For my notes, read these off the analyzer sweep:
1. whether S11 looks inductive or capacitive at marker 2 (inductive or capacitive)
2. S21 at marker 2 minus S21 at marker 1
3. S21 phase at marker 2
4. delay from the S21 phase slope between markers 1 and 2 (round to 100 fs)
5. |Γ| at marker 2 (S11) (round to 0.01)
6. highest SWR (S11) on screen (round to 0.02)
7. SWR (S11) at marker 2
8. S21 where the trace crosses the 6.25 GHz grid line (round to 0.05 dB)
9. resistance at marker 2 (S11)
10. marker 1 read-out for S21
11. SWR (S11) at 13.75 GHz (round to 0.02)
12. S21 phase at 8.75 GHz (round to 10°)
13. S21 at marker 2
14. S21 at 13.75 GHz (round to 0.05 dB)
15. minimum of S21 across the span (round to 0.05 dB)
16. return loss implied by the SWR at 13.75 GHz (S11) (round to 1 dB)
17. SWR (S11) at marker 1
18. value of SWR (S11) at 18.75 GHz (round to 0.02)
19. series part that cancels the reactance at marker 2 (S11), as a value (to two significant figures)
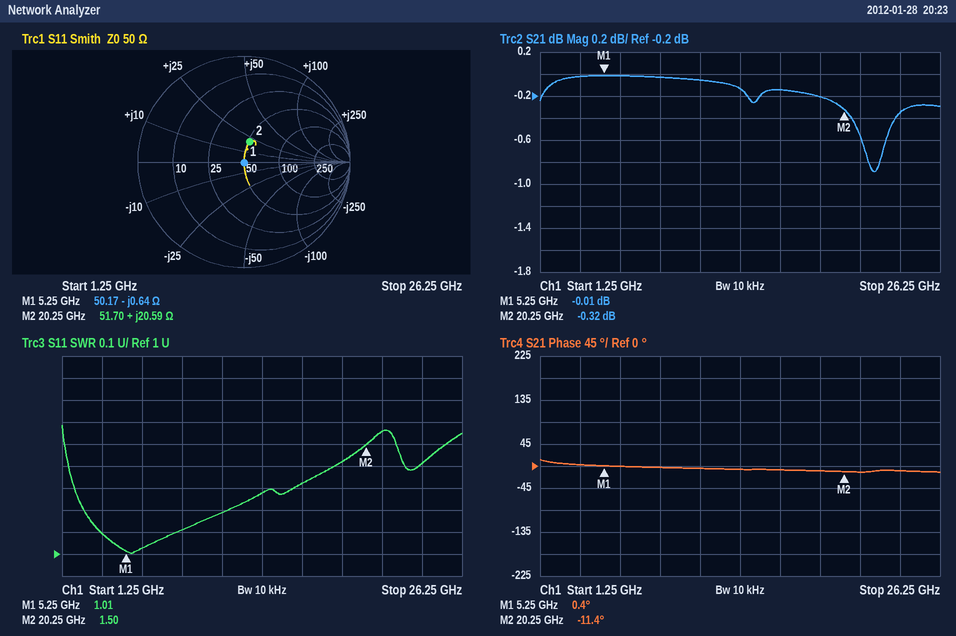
inductive
-0.31 dB
-11.4°
2.2 ps
0.20
1.58
1.50
0.00 dB
51.70 Ω
-0.01 dB
1.28
0°
-0.32 dB
-0.15 dB
-0.90 dB
18 dB
1.01
1.42
380 fF
